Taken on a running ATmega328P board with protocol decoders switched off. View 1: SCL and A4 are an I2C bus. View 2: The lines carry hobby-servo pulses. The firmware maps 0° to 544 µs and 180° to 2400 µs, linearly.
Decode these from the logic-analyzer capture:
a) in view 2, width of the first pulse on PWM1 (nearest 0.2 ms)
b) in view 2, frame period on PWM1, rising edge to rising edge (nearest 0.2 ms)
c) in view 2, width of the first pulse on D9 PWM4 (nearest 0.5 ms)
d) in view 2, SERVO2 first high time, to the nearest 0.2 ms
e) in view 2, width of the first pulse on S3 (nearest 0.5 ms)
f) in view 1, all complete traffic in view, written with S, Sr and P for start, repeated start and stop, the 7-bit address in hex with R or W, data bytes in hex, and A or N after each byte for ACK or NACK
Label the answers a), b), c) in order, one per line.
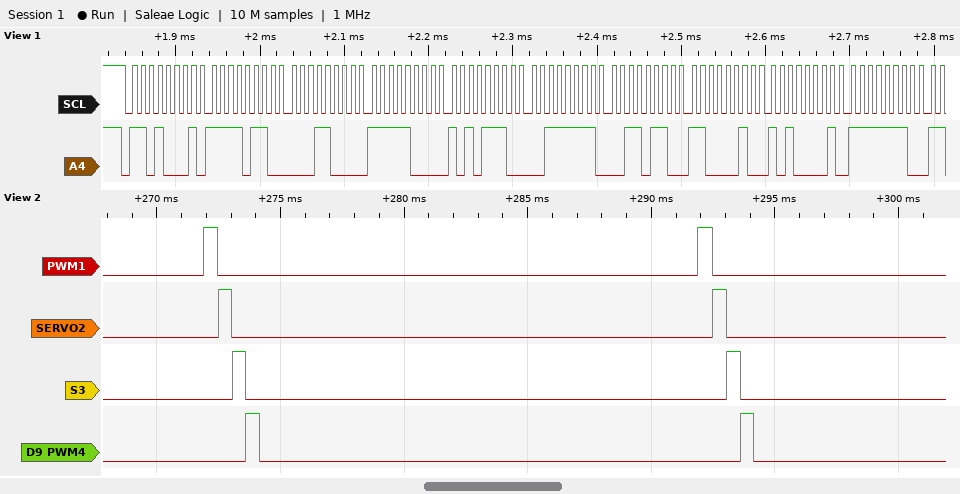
a) 0.6 ms
b) 20.0 ms
c) 0.5 ms
d) 0.6 ms
e) 0.5 ms
f) S 68R A F6 A 18 A F8 A AE A 3F A 36 A C2 A A1 A FE A
